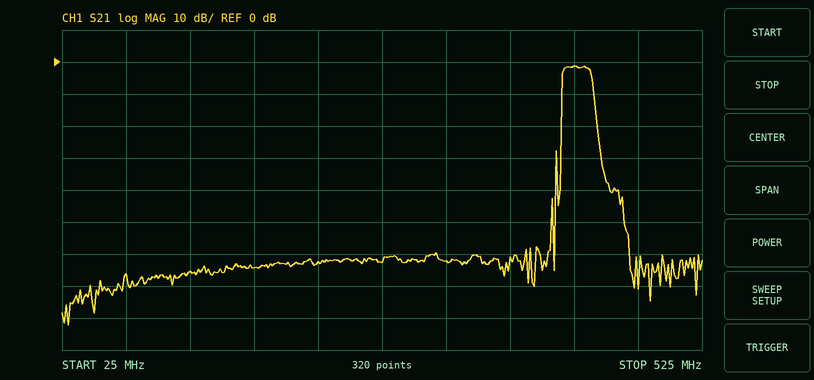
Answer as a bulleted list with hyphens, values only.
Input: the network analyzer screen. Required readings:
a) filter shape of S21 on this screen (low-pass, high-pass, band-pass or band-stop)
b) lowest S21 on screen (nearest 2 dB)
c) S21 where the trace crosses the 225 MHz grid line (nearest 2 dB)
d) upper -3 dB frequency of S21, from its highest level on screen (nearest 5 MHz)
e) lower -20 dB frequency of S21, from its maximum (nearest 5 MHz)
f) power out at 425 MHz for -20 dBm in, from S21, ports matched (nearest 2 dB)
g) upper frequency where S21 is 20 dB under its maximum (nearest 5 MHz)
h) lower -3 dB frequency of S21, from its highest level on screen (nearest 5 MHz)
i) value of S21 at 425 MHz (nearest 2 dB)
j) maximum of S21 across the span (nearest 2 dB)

- band-pass
- -82 dB
- -62 dB
- 440 MHz
- 415 MHz
- -22 dBm
- 445 MHz
- 415 MHz
- -2 dB
- -2 dB
